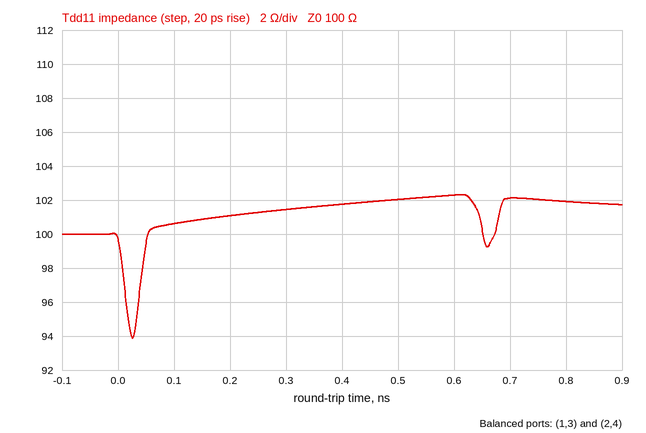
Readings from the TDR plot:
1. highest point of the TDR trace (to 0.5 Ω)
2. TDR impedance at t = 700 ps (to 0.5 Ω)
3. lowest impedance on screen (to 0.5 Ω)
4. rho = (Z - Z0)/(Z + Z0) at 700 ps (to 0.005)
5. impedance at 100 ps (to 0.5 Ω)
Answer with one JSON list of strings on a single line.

["102.5 Ω", "102.0 Ω", "94.0 Ω", "+0.010", "100.5 Ω"]
